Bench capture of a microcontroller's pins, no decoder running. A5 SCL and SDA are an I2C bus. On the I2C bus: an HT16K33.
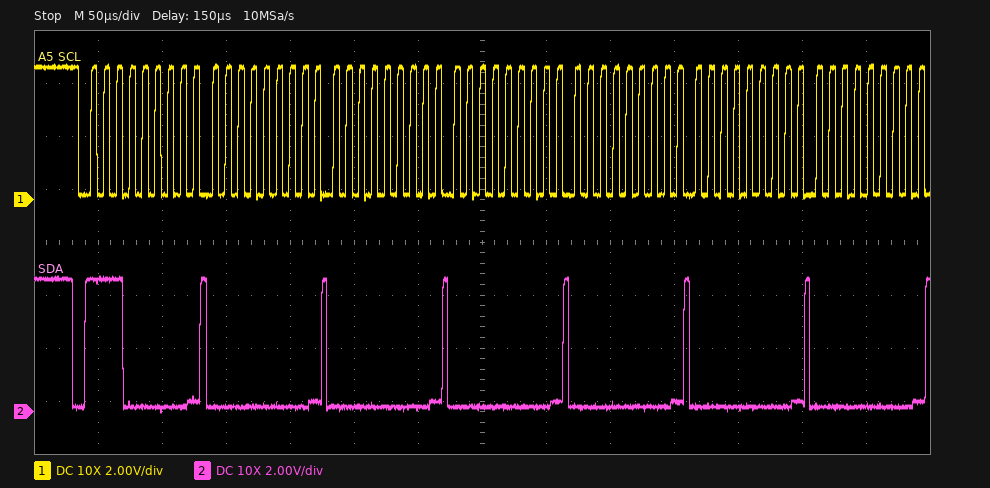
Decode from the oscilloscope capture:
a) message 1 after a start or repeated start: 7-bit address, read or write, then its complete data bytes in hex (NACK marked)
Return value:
0x70 write: 00 00 00 00 00 00
